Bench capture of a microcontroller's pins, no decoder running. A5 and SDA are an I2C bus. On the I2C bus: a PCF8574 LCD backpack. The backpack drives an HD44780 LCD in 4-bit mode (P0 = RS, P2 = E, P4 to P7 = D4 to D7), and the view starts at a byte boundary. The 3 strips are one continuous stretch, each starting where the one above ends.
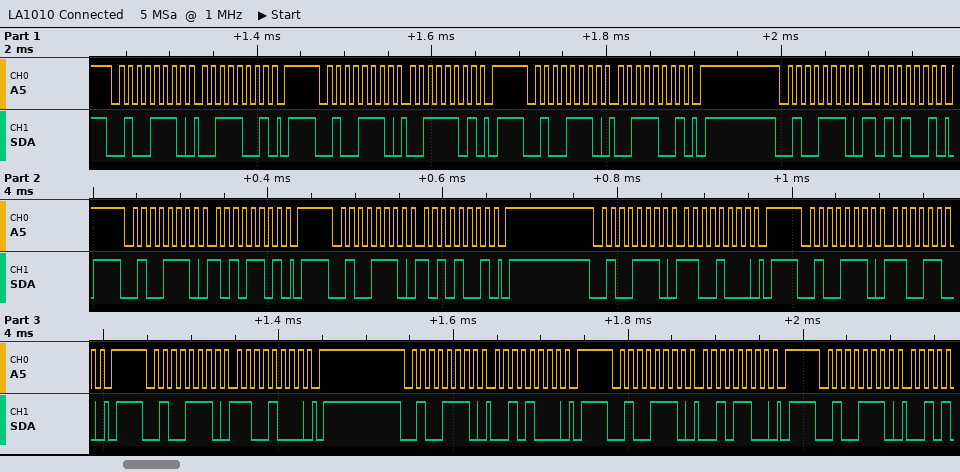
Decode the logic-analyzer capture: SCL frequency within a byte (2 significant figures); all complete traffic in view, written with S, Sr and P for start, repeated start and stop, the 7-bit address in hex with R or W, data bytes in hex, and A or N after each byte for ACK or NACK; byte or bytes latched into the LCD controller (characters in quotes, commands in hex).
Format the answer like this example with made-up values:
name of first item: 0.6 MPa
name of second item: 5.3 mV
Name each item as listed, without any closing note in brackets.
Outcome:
SCL frequency within a byte: 100 kHz
all complete traffic in view, written with S, Sr and P for start, repeated start and stop, the 7-bit address in hex with R or W, data bytes in hex, and A or N after each byte for ACK or NACK: S 27W A 39 A P S 27W A 3D A P S 27W A 39 A P S 27W A A9 A P S 27W A AD A P S 27W A A9 A P S 27W A C8 A P S 27W A CC A P S 27W A C8 A P S 27W A 28 A P S 27W A 2C A P S 27W A
byte or bytes latched into the LCD controller: ':'
